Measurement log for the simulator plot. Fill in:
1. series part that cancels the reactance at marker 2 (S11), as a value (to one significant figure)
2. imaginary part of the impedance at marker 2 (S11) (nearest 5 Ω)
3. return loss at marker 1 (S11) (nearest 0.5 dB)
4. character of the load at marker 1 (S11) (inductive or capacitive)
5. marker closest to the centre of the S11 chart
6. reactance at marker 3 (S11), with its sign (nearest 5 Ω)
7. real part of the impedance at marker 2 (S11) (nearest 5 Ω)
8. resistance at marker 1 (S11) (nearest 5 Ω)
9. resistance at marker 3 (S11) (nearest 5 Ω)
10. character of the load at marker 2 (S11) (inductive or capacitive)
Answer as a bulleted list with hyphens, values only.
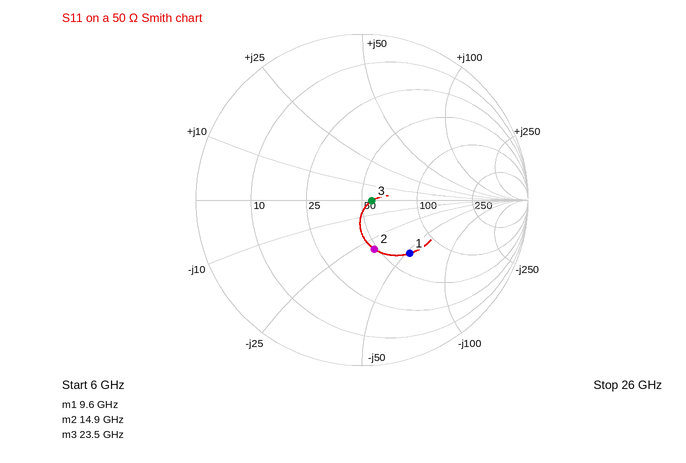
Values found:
- 300 pH
- -30 Ω
- 7.5 dB
- capacitive
- marker 3
- 0 Ω
- 50 Ω
- 65 Ω
- 55 Ω
- capacitive
